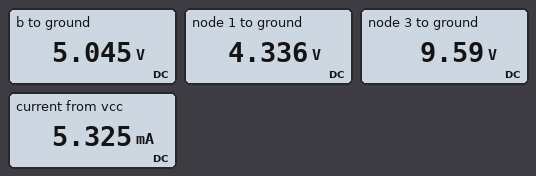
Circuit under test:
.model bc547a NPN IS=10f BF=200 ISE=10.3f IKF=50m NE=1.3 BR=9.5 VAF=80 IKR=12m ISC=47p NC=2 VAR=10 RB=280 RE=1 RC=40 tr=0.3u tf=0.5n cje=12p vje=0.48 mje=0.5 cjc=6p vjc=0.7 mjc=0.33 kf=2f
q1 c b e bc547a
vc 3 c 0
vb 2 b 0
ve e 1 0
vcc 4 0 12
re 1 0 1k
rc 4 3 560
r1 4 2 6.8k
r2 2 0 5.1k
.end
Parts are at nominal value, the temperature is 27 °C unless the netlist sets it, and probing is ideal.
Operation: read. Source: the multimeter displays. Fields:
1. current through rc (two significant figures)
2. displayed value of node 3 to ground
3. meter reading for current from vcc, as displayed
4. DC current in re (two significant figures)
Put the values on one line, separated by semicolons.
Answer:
4.3 mA; 9.59 V; 5.325 mA; 4.3 mA
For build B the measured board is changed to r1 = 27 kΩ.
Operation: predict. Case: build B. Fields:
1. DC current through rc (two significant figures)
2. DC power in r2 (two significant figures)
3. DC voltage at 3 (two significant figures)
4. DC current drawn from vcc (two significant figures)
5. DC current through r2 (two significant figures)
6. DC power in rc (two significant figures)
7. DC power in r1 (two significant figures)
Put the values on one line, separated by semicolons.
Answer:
1.2 mA; 680 µW; 11 V; 1.6 mA; 370 µA; 800 µW; 3.8 mW
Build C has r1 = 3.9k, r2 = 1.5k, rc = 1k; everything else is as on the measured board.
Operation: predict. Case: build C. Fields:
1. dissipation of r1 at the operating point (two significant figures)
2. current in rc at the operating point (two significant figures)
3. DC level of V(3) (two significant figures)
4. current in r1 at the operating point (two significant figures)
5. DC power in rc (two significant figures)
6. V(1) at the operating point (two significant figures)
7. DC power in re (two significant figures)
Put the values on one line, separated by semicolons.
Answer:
19 mW; 2.6 mA; 9.4 V; 2.2 mA; 6.8 mW; 2.6 V; 6.9 mW
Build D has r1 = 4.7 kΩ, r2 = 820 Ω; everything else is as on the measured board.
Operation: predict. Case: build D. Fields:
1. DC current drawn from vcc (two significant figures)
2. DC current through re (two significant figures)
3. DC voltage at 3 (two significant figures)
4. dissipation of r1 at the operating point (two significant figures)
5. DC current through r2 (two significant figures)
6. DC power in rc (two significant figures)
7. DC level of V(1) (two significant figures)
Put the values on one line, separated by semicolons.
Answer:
3.3 mA; 1.1 mA; 11 V; 22 mW; 2.2 mA; 690 µW; 1.1 V
